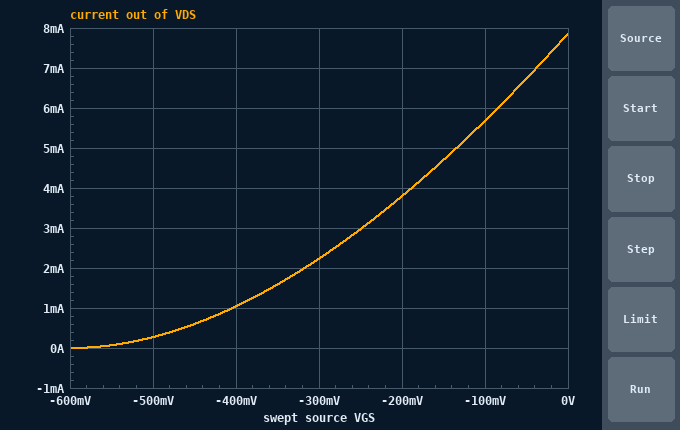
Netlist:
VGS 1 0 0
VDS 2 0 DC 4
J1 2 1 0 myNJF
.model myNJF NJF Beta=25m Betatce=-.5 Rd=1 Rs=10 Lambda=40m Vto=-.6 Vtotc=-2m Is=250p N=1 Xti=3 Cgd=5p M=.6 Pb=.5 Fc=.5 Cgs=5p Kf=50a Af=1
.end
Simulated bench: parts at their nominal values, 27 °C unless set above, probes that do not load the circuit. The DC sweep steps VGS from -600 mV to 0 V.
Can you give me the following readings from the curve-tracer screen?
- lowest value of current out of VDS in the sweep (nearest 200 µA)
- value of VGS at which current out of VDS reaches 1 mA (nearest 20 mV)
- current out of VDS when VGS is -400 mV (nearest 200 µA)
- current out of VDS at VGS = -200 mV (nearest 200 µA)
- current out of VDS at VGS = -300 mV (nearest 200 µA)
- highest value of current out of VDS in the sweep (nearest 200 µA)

0 A
-400 mV
1.0 mA
3.8 mA
2.2 mA
7.8 mA
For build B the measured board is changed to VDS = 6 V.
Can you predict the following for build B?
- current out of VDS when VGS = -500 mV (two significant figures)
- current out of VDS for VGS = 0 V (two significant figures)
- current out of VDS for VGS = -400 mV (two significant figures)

290 µA
8.3 mA
1.1 mA
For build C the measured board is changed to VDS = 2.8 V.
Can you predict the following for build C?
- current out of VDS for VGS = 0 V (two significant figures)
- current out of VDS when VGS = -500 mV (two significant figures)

7.6 mA
260 µA
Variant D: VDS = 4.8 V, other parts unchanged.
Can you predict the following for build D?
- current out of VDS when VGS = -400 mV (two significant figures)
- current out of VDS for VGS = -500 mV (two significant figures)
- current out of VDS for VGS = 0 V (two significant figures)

1.1 mA
280 µA
8.0 mA
